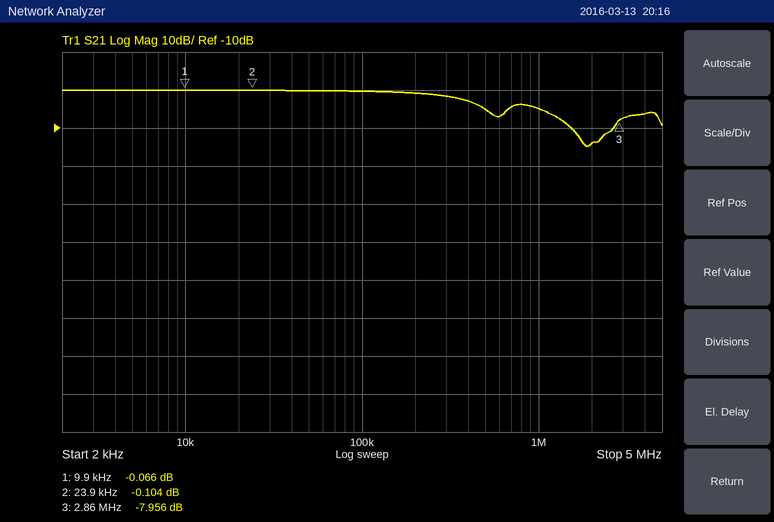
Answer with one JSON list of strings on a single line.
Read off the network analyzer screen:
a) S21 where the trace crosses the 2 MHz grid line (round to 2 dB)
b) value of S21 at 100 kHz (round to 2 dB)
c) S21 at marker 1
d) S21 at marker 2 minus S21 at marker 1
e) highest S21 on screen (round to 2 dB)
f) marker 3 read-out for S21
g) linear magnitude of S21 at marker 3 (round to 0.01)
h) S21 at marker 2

["-14 dB", "0 dB", "-0.066 dB", "-0.038 dB", "0 dB", "-7.956 dB", "0.40", "-0.104 dB"]
